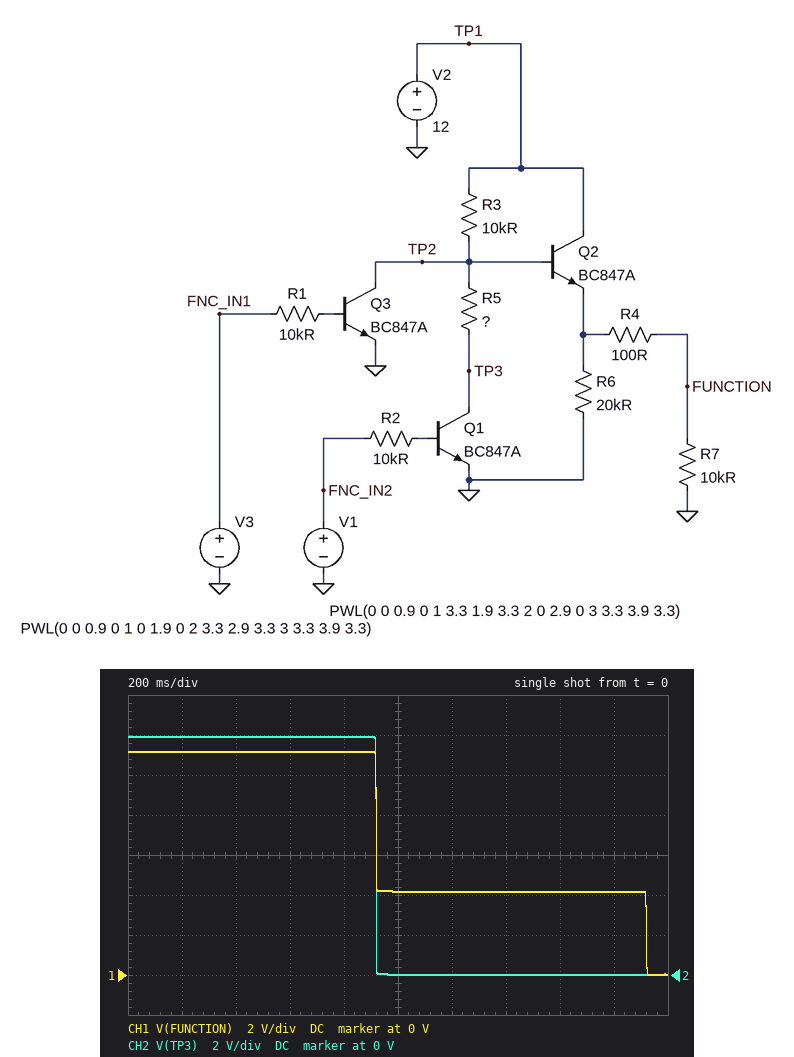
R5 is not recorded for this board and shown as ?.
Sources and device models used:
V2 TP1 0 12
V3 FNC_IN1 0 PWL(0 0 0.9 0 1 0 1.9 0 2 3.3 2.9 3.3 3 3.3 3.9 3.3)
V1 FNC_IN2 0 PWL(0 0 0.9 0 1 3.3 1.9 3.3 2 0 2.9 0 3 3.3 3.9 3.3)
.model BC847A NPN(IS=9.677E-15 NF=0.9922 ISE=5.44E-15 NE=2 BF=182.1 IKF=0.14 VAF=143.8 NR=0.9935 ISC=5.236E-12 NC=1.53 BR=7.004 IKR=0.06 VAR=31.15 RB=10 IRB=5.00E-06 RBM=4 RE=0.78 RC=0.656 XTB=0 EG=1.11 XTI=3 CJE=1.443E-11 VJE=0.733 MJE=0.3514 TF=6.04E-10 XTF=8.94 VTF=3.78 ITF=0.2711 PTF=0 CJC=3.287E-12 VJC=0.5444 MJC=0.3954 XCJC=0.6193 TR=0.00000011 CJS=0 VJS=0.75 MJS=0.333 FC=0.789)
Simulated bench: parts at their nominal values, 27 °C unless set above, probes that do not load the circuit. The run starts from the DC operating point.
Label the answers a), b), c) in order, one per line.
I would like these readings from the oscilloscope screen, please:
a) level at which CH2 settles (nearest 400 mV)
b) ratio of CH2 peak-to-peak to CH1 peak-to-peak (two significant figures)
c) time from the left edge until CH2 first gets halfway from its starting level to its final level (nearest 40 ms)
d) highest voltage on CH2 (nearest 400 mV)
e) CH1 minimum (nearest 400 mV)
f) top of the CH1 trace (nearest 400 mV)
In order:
a) 0 V
b) 1.1
c) 920 ms
d) 12.0 V
e) 0 V
f) 11.2 V
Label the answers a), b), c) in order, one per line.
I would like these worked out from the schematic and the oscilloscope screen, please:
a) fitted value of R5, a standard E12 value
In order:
a) 6.8 kΩ
